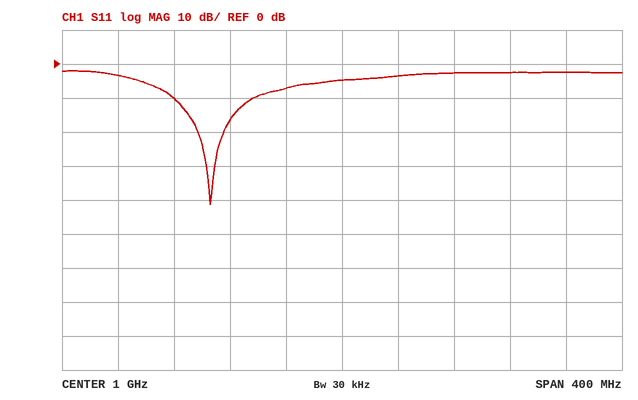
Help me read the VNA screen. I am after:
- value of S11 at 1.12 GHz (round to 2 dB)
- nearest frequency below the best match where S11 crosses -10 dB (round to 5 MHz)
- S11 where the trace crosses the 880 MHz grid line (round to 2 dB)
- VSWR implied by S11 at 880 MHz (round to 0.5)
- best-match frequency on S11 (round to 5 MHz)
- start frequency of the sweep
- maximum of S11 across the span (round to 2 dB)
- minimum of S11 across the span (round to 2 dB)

-2 dB
880 MHz
-10 dB
2.0
905 MHz
800 MHz
-2 dB
-42 dB
